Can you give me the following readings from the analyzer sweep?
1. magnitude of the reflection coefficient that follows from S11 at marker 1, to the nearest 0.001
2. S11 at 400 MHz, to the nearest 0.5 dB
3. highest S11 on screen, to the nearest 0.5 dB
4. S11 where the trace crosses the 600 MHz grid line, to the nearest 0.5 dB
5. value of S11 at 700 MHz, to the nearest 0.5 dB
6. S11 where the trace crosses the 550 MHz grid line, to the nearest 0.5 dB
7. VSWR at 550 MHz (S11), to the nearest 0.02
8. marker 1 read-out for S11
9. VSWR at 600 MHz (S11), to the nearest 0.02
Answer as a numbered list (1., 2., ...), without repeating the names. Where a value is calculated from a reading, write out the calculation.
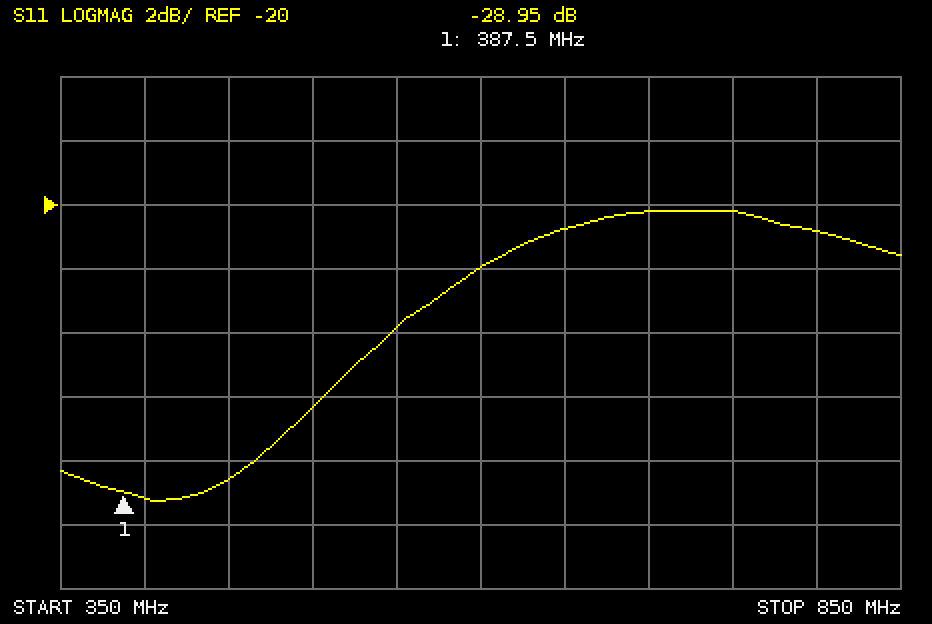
1. 10^(-28.95/20) ≈ 0.036
2. -29.0 dB
3. -20.0 dB
4. -22.0 dB
5. -20.0 dB
6. -24.0 dB
7. |Γ| = 10^(-24/20) = 0.0631; VSWR = (1 + 0.0631)/(1 − 0.0631) ≈ 1.13, so 1.14 to the nearest 0.02
8. -28.95 dB
9. |Γ| = 10^(-22/20) = 0.0794; VSWR = (1 + 0.0794)/(1 − 0.0794) ≈ 1.17, so 1.18 to the nearest 0.02
